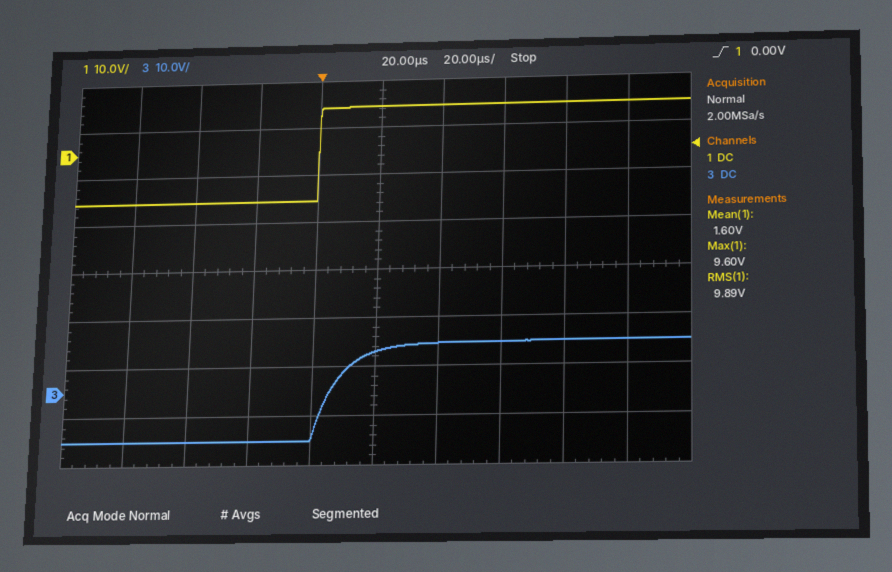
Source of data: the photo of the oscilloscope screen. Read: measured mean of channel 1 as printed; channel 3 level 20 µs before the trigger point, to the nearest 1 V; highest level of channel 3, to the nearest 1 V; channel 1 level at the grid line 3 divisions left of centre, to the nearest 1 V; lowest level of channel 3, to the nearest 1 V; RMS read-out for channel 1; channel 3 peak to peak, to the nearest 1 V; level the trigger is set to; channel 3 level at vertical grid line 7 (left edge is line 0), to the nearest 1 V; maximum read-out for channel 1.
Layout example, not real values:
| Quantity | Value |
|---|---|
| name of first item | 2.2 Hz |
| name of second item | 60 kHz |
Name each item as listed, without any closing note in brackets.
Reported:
| Quantity | Value |
|---|---|
| measured mean of channel 1 as printed | 1.60 V |
| channel 3 level 20 µs before the trigger point, to the nearest 1 V | -10 V |
| highest level of channel 3, to the nearest 1 V | 10 V |
| channel 1 level at the grid line 3 divisions left of centre, to the nearest 1 V | -10 V |
| lowest level of channel 3, to the nearest 1 V | -10 V |
| RMS read-out for channel 1 | 9.89 V |
| channel 3 peak to peak, to the nearest 1 V | 20 V |
| level the trigger is set to | 0.00 V |
| channel 3 level at vertical grid line 7 (left edge is line 0), to the nearest 1 V | 10 V |
| maximum read-out for channel 1 | 9.60 V |
